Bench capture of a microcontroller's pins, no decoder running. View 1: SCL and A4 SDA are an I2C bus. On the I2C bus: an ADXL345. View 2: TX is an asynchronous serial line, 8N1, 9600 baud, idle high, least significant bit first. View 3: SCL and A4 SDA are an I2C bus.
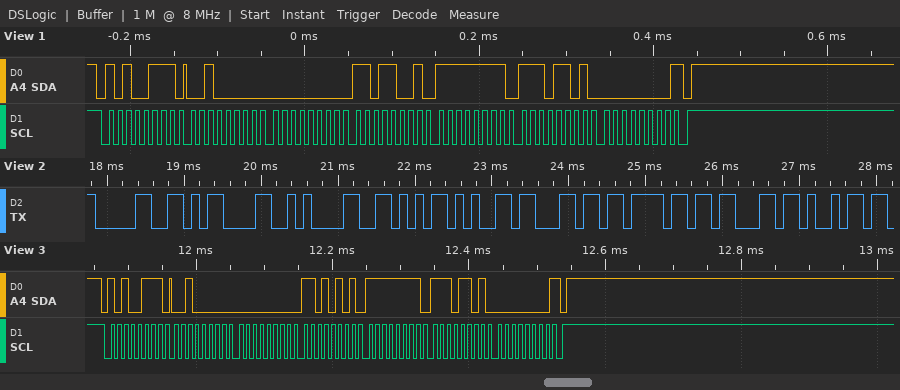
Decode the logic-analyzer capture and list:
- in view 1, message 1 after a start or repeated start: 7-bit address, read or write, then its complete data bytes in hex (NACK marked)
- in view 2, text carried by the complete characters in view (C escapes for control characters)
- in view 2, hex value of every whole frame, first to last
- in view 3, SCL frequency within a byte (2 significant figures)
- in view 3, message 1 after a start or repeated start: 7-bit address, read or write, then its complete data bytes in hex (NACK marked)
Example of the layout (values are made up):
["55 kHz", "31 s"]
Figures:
["0x53 read: 20 00 D9 FF ED 00 NACK", "\"0\\r\\nVeloci\"", "30 0D 0A 56 65 6C 6F 63 69", "100 kHz", "0x53 read: 20 00 D5 FF ED 00 NACK"]
